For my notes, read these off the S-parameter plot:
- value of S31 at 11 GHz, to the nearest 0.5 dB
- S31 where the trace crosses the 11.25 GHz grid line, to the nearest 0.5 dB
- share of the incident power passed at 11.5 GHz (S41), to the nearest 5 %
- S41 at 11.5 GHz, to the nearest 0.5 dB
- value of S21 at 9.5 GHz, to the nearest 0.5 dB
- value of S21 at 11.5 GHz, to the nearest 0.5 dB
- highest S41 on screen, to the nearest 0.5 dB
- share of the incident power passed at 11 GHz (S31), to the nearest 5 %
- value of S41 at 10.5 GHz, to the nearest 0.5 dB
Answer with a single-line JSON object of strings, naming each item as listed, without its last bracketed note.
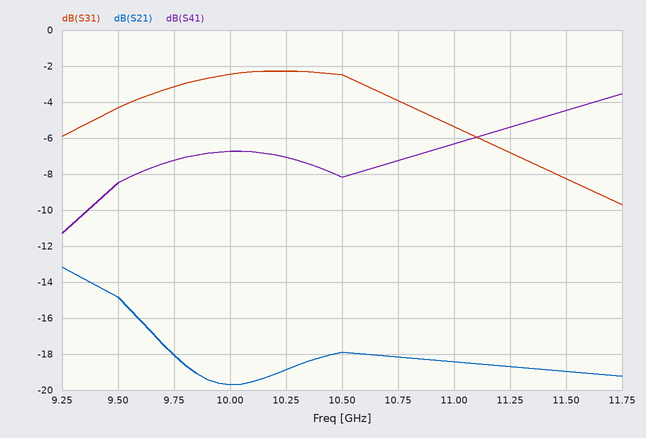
{"value of S31 at 11 GHz, to the nearest 0.5 dB": "-5.5 dB", "S31 where the trace crosses the 11.25 GHz grid line, to the nearest 0.5 dB": "-7.0 dB", "share of the incident power passed at 11.5 GHz (S41), to the nearest 5 %": "35 %", "S41 at 11.5 GHz, to the nearest 0.5 dB": "-4.5 dB", "value of S21 at 9.5 GHz, to the nearest 0.5 dB": "-15.0 dB", "value of S21 at 11.5 GHz, to the nearest 0.5 dB": "-19.0 dB", "highest S41 on screen, to the nearest 0.5 dB": "-3.5 dB", "share of the incident power passed at 11 GHz (S31), to the nearest 5 %": "30 %", "value of S41 at 10.5 GHz, to the nearest 0.5 dB": "-8.0 dB"}
